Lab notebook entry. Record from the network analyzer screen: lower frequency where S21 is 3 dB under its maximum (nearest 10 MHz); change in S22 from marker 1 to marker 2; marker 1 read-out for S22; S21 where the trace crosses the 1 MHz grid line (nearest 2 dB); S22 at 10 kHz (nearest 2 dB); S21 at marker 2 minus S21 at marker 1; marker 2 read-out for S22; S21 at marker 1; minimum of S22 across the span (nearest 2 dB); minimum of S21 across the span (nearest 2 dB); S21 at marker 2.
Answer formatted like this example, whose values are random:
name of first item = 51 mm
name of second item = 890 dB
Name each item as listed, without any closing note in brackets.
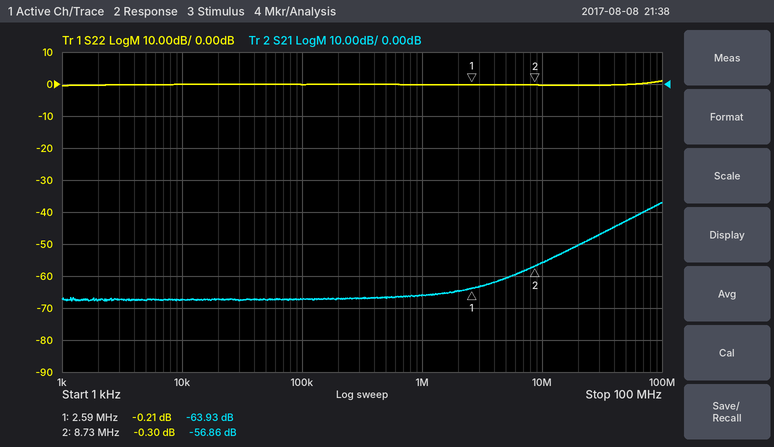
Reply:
lower frequency where S21 is 3 dB under its maximum = 70 MHz
change in S22 from marker 1 to marker 2 = -0.09 dB
marker 1 read-out for S22 = -0.21 dB
S21 where the trace crosses the 1 MHz grid line = -66 dB
S22 at 10 kHz = 0 dB
S21 at marker 2 minus S21 at marker 1 = 7.07 dB
marker 2 read-out for S22 = -0.30 dB
S21 at marker 1 = -63.93 dB
minimum of S22 across the span = 0 dB
minimum of S21 across the span = -68 dB
S21 at marker 2 = -56.86 dB
